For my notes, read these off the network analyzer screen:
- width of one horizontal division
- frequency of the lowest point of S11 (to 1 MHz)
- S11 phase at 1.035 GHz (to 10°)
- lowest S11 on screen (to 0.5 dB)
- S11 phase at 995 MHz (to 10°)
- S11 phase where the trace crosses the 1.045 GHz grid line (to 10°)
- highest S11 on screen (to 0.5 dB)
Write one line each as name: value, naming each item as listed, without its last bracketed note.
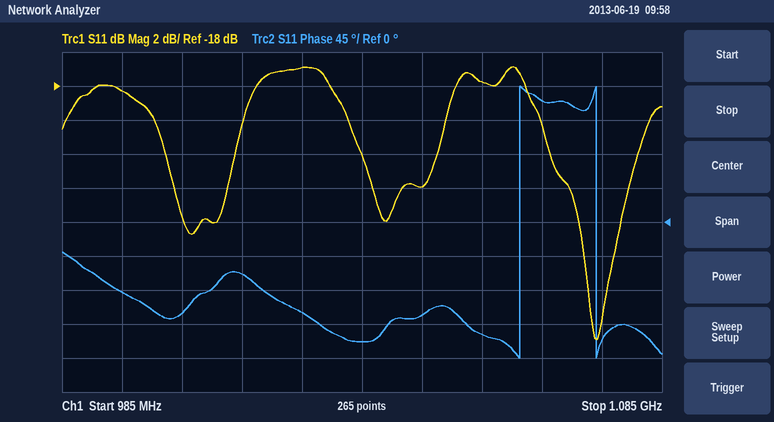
width of one horizontal division: 10 MHz
frequency of the lowest point of S11: 1.074 GHz
S11 phase at 1.035 GHz: -160°
lowest S11 on screen: -33.0 dB
S11 phase at 995 MHz: -90°
S11 phase where the trace crosses the 1.045 GHz grid line: -120°
highest S11 on screen: -17.0 dB
